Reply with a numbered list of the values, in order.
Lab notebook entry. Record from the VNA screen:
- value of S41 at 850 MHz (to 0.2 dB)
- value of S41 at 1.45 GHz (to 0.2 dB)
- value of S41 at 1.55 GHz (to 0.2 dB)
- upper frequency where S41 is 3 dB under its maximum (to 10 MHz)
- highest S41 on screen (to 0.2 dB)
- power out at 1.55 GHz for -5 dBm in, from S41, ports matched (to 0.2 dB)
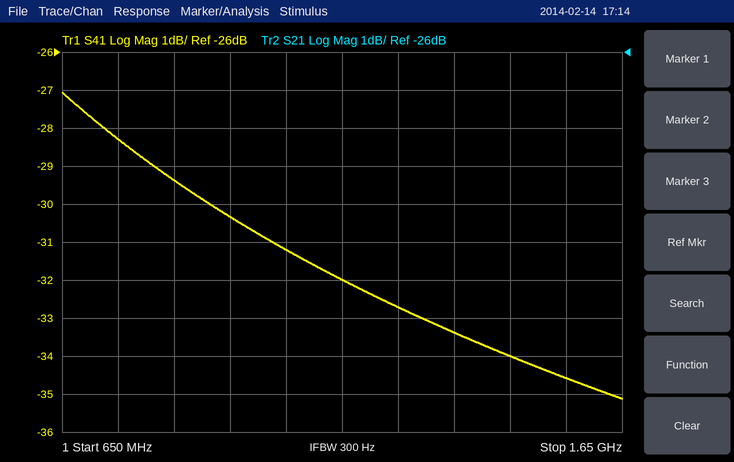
1. -29.4 dB
2. -34.0 dB
3. -34.6 dB
4. 920 MHz
5. -27.0 dB
6. -39.6 dBm
